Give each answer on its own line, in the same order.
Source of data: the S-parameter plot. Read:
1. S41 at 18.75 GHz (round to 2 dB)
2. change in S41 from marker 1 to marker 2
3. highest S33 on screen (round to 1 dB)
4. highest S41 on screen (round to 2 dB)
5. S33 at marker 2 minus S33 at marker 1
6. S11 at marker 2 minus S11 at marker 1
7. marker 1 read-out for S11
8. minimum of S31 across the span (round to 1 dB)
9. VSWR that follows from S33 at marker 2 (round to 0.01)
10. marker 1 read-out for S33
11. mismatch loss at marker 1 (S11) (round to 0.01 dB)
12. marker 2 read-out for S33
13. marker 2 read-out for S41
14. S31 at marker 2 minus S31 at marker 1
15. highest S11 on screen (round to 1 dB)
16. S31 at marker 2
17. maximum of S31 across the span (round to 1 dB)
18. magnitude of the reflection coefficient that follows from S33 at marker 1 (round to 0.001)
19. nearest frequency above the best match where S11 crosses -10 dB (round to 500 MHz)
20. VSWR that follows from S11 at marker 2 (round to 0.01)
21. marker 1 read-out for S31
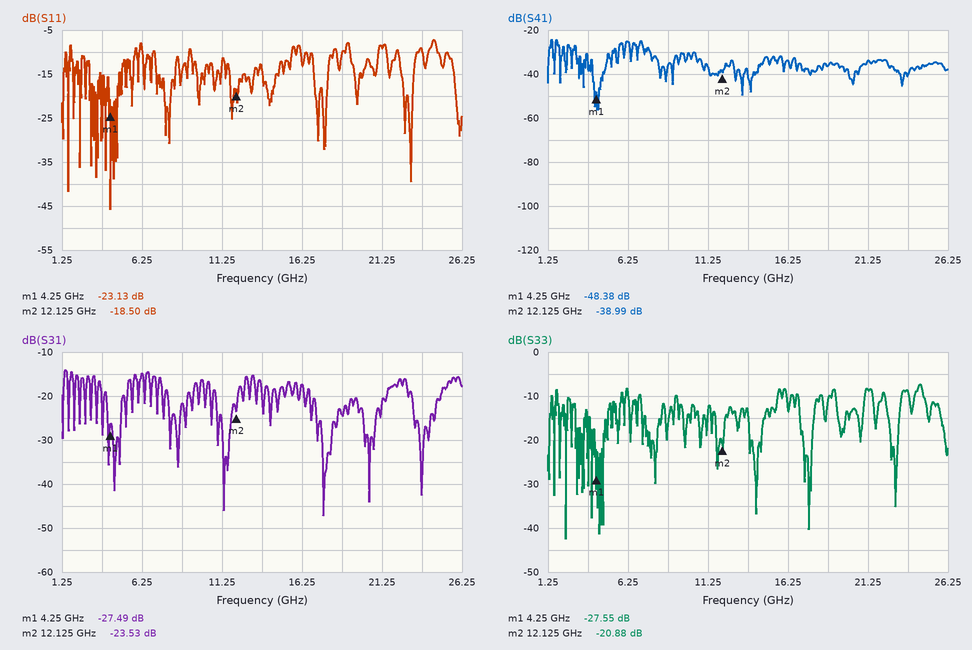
-36 dB
9.39 dB
-7 dB
-24 dB
6.67 dB
4.63 dB
-23.13 dB
-47 dB
1.20
-27.55 dB
0.02 dB
-20.88 dB
-38.99 dB
3.96 dB
-7 dB
-23.53 dB
-14 dB
0.042
6.0 GHz
1.27
-27.49 dB
